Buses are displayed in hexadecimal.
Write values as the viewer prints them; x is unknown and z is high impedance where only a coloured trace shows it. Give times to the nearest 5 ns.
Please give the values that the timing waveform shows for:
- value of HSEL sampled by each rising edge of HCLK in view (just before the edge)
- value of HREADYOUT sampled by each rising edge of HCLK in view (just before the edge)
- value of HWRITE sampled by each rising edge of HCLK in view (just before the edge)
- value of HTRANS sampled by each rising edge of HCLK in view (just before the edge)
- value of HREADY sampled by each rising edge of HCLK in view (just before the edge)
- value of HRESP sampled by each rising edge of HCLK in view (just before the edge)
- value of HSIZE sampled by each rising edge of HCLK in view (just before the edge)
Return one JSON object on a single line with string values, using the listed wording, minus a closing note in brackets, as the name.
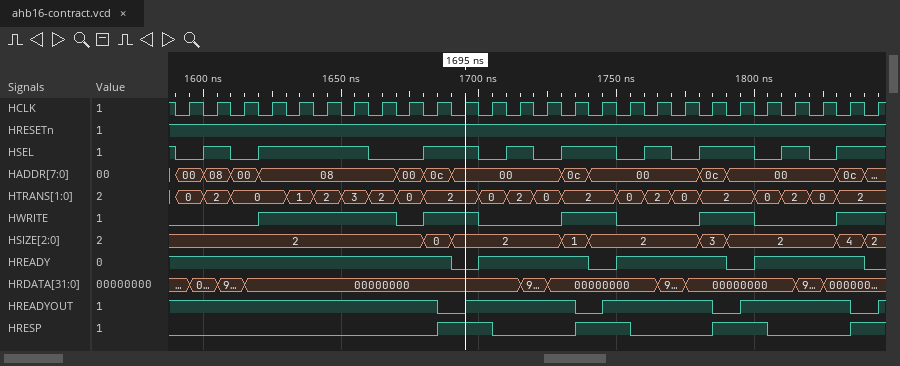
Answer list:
{"value of HSEL sampled by each rising edge of HCLK in view": "0 1 0 1 1 1 1 0 0 1 1 0 1 0 1 1 0 1 0 1 1 0 1 0 1 1", "value of HREADYOUT sampled by each rising edge of HCLK in view": "1 1 1 1 1 1 1 1 1 1 0 1 1 1 1 0 1 1 1 1 0 1 1 1 1 0", "value of HWRITE sampled by each rising edge of HCLK in view": "0 0 0 1 1 1 1 1 0 1 1 0 0 0 1 1 0 0 0 1 1 0 0 0 1 1", "value of HTRANS sampled by each rising edge of HCLK in view": "0, 2, 0, 0, 1, 2, 3, 2, 0, 2, 2, 0, 2, 0, 2, 2, 0, 2, 0, 2, 2, 0, 2, 0, 2, 2", "value of HREADY sampled by each rising edge of HCLK in view": "1 1 1 1 1 1 1 1 1 1 0 1 1 1 1 0 1 1 1 1 0 1 1 1 1 0", "value of HRESP sampled by each rising edge of HCLK in view": "0 0 0 0 0 0 0 0 0 0 1 1 0 0 0 1 1 0 0 0 1 1 0 0 0 1", "value of HSIZE sampled by each rising edge of HCLK in view": "2, 2, 2, 2, 2, 2, 2, 2, 2, 0, 2, 2, 2, 2, 1, 2, 2, 2, 2, 3, 2, 2, 2, 2, 4, 2"}
